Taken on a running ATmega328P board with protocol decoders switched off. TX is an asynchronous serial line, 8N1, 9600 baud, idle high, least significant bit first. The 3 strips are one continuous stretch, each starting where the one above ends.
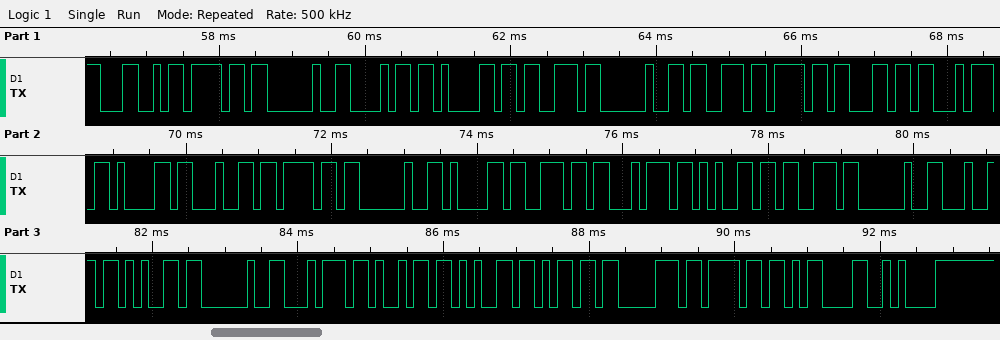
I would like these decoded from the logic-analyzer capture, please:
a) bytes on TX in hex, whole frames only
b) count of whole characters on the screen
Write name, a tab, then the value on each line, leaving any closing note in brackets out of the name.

bytes on TX in hex, whole frames only	4C 6F 20 68 61 73 20 73 6F 6C 74 61 64 6F 20 61 6E 74 65 73 20 64 65 20 74 69 65 6D 70 6F 0D 0A
count of whole characters on the screen	32
